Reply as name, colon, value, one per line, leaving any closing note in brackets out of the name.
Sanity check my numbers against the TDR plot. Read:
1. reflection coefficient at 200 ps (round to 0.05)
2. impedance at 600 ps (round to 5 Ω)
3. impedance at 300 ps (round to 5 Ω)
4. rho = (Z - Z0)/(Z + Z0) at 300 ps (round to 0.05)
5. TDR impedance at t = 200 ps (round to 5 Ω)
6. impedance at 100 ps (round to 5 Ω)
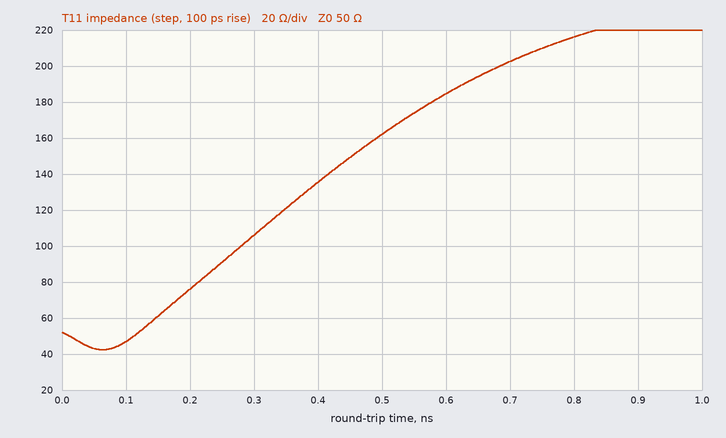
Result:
reflection coefficient at 200 ps: +0.20
impedance at 600 ps: 185 Ω
impedance at 300 ps: 105 Ω
rho = (Z - Z0)/(Z + Z0) at 300 ps: +0.35
TDR impedance at t = 200 ps: 75 Ω
impedance at 100 ps: 45 Ω
